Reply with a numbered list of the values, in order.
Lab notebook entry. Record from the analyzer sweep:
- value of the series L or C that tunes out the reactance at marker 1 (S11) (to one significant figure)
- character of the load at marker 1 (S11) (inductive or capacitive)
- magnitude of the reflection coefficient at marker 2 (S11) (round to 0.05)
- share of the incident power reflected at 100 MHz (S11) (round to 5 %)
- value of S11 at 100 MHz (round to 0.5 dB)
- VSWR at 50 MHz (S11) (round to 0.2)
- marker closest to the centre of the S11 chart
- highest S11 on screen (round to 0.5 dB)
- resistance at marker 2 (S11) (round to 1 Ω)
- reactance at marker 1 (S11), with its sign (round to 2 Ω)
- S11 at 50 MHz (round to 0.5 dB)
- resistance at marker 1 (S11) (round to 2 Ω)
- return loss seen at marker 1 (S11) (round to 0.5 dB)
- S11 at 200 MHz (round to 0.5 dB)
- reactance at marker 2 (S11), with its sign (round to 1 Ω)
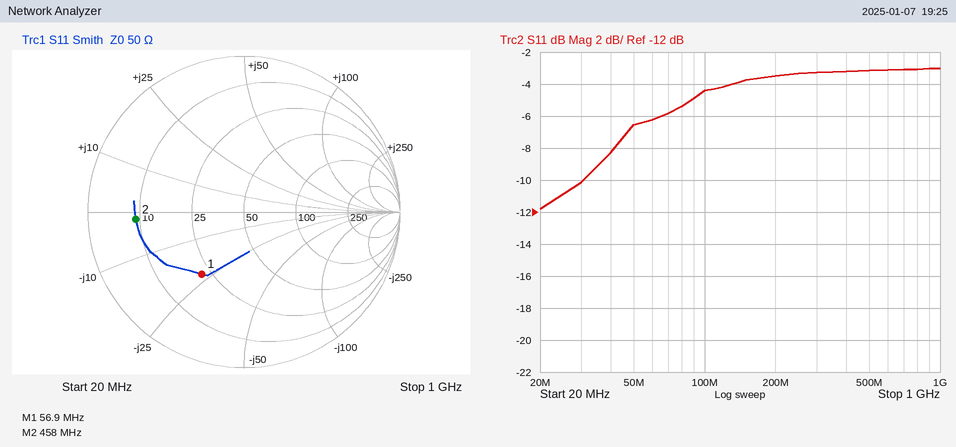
1. 60 nH
2. capacitive
3. 0.70
4. 35 %
5. -4.5 dB
6. 2.8
7. marker 1
8. -3.0 dB
9. 9 Ω
10. -22 Ω
11. -6.5 dB
12. 22 Ω
13. 6.5 dB
14. -3.5 dB
15. -2 Ω
